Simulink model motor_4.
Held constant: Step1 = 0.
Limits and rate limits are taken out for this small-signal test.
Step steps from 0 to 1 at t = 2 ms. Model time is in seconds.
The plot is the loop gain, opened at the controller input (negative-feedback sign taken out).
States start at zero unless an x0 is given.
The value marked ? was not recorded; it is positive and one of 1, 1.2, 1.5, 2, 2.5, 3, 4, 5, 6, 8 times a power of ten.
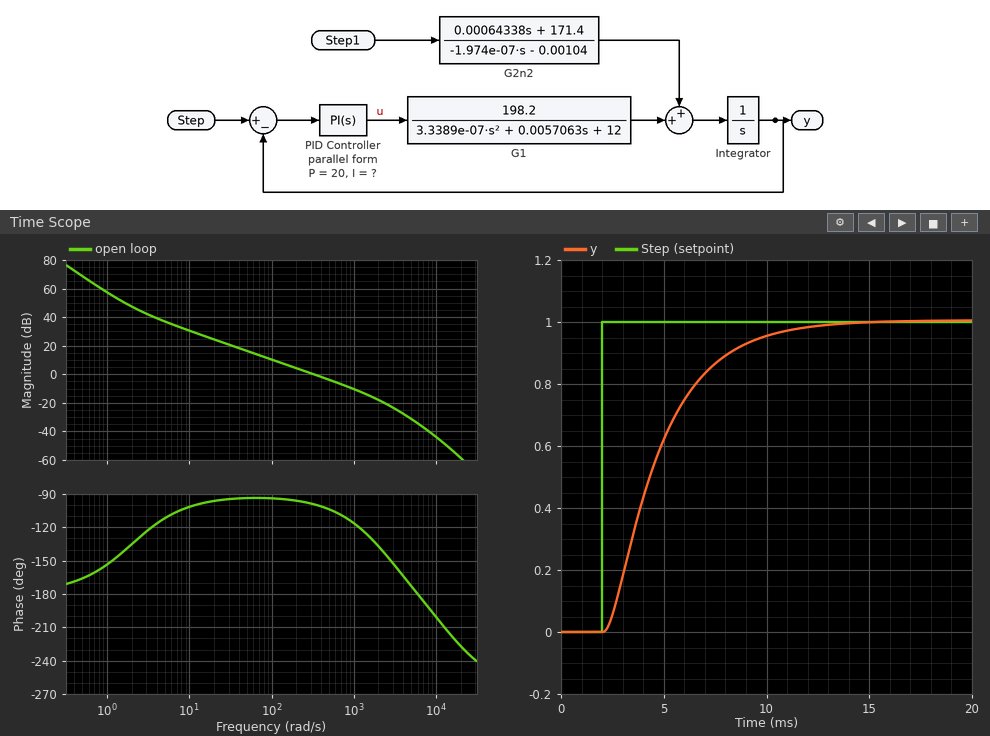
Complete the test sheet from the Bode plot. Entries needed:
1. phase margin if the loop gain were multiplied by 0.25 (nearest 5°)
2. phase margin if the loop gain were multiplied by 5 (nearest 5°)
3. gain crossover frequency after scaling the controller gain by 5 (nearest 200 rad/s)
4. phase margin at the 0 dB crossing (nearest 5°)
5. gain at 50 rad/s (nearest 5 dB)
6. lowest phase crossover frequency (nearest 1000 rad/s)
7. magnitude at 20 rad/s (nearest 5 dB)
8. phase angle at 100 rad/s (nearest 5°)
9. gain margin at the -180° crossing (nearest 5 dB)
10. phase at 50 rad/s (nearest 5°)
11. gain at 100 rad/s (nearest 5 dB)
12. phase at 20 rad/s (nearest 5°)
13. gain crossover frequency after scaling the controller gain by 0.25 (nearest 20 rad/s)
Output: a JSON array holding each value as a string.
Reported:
["85°", "55°", "1400 rad/s", "80°", "15 dB", "6000 rad/s", "25 dB", "-95°", "35 dB", "-95°", "10 dB", "-95°", "80 rad/s"]
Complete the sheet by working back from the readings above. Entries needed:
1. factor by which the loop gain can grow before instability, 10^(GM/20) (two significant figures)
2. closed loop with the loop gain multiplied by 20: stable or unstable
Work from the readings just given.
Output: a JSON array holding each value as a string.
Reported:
["56", "stable"]
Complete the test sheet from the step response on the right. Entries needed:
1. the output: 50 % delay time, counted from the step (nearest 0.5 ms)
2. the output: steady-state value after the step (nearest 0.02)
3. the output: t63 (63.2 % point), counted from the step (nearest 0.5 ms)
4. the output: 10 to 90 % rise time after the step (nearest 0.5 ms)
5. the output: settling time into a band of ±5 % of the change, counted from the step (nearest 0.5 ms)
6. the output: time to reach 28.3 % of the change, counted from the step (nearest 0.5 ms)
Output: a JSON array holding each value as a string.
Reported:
["2.5 ms", "1.00", "3.0 ms", "5.5 ms", "8.0 ms", "1.5 ms"]
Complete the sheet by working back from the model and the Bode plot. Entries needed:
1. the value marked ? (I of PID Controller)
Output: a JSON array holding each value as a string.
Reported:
["40"]
